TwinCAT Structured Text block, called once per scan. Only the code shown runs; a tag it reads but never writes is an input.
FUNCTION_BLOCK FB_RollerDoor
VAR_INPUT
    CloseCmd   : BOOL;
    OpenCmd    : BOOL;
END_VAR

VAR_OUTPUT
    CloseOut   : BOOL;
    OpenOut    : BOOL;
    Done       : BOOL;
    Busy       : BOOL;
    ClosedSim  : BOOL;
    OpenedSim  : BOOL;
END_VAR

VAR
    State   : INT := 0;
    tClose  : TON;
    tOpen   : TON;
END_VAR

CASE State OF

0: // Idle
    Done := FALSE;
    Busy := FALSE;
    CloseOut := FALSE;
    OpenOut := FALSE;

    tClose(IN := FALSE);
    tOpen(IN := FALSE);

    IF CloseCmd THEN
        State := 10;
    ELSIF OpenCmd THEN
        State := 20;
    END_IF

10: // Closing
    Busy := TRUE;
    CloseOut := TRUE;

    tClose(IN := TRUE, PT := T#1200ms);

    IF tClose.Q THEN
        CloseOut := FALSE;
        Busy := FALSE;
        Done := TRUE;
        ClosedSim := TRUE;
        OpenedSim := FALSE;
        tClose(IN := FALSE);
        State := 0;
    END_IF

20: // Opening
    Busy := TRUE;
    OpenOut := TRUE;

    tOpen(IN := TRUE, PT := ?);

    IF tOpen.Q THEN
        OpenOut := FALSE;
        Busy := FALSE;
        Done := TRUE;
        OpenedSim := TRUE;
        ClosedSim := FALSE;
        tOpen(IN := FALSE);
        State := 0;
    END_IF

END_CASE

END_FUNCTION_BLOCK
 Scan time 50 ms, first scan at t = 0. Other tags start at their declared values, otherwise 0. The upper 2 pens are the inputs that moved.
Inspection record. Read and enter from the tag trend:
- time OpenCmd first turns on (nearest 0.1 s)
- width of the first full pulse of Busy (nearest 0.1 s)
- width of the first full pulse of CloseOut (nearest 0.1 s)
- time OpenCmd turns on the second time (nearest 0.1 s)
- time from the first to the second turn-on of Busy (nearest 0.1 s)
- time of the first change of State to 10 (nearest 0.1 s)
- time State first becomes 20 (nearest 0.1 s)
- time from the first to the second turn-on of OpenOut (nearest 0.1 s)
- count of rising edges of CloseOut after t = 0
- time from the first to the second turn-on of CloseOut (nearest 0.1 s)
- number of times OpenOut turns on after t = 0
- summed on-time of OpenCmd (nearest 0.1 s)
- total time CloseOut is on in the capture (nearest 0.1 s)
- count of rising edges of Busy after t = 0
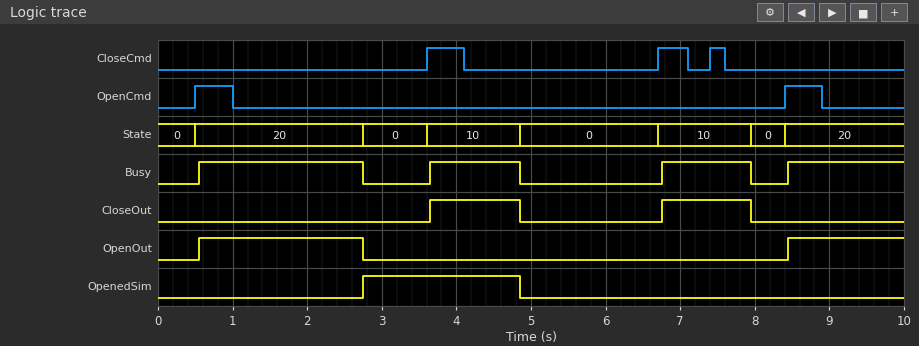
0.5 s
2.2 s
1.2 s
8.4 s
3.1 s
3.6 s
0.5 s
7.9 s
2
3.1 s
2
1.0 s
2.4 s
4
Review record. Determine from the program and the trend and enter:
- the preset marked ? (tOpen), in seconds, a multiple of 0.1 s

2.2 s
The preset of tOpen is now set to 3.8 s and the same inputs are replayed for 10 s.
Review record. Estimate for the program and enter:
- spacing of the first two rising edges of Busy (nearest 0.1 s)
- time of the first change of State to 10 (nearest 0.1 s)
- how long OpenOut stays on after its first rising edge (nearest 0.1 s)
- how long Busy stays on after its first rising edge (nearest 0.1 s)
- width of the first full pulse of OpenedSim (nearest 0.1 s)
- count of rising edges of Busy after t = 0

6.2 s
6.7 s
3.8 s
3.8 s
3.6 s
3
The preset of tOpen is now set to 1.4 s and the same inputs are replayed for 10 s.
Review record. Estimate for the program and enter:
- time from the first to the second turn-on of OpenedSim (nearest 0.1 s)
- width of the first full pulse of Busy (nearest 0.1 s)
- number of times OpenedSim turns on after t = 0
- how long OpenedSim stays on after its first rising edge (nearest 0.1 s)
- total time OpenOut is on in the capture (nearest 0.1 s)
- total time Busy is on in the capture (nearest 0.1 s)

7.9 s
1.4 s
2
2.9 s
2.8 s
5.2 s
